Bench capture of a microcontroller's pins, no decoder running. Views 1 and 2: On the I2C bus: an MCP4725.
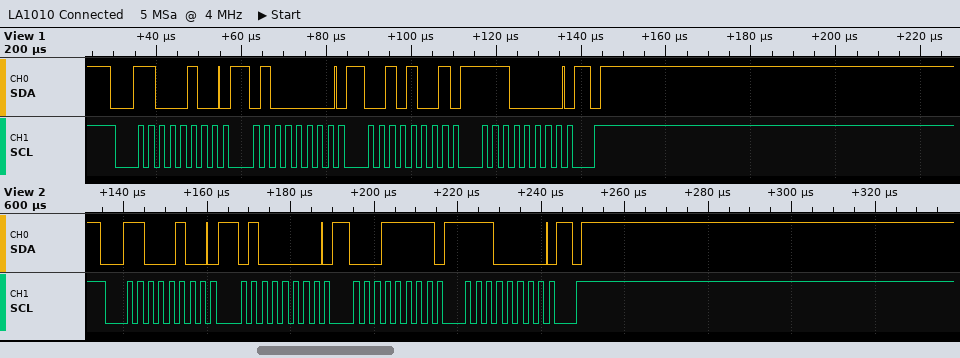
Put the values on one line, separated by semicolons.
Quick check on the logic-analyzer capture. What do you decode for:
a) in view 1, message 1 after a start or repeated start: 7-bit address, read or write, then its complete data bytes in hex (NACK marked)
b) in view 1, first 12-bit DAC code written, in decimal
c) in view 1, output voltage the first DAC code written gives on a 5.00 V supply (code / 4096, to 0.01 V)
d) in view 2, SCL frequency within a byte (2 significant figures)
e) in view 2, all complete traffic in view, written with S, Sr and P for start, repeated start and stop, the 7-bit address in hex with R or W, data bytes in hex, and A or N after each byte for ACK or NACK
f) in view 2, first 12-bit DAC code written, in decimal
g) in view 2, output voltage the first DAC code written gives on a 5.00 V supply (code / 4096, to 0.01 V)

0x62 write: 40 29 E0; 670; 0.82 V; 400 kHz; S 62W A 40 A 1F A E0 A P; 510; 0.62 V
